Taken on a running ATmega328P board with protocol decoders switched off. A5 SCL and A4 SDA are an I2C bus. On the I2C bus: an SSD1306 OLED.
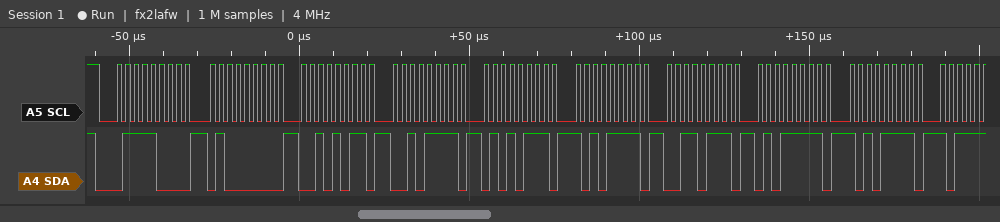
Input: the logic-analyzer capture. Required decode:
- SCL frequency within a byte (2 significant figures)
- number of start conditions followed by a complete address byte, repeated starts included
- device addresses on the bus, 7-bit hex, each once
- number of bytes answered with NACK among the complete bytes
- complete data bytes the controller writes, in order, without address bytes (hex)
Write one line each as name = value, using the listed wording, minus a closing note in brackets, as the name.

SCL frequency within a byte = 400 kHz
number of start conditions followed by a complete address byte, repeated starts included = 1
device addresses on the bus, 7-bit hex, each once = 0x3C
number of bytes answered with NACK among the complete bytes = 0
complete data bytes the controller writes, in order, without address bytes = 40 2B 2F 57 AF 37 5F AF
